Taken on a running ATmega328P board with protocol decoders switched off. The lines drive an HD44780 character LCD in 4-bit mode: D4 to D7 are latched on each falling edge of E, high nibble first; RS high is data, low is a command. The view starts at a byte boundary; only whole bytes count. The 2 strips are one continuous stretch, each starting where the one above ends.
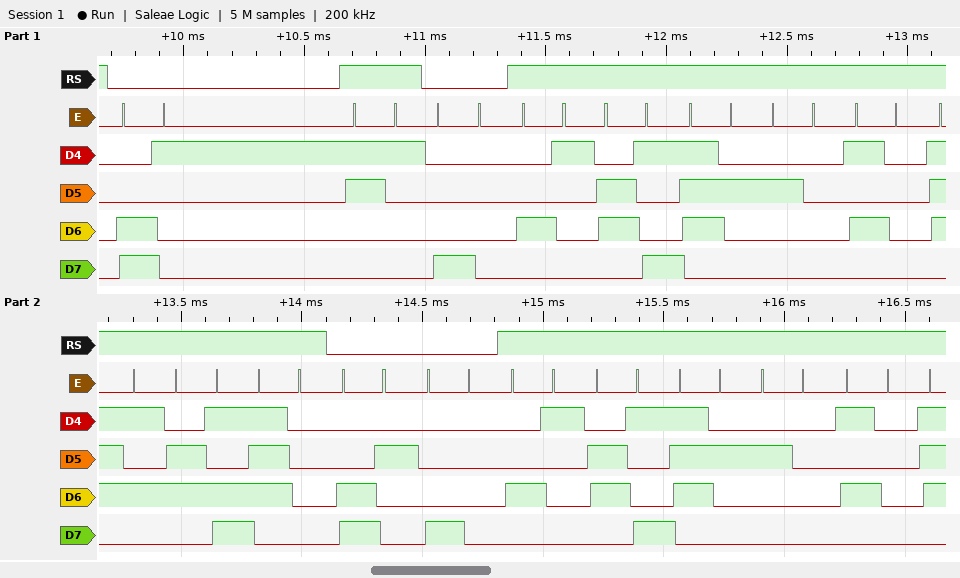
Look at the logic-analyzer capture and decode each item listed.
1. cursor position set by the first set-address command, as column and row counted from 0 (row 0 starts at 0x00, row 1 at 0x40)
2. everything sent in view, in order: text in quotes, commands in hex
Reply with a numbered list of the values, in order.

1. column 1, row 1
2. 0xC1 "1" 0x80 "Air Pump" 0xC2 0x80 "Air P"
